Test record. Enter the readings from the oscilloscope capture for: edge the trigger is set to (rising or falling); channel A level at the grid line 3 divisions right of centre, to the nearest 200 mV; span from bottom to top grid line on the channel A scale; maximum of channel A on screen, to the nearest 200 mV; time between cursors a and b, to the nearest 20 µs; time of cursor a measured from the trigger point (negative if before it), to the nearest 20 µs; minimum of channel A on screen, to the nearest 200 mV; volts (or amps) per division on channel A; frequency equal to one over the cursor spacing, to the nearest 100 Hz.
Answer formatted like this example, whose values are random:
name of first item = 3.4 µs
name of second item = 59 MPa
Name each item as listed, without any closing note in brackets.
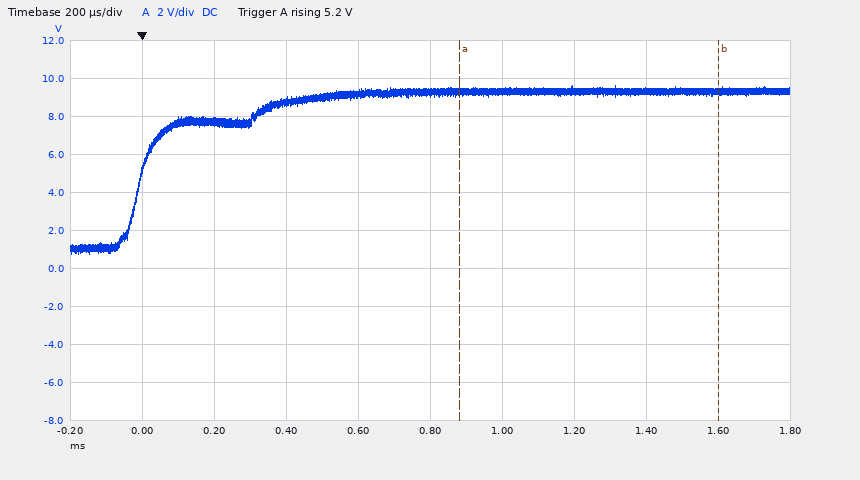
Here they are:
edge the trigger is set to = rising
channel A level at the grid line 3 divisions right of centre, to the nearest 200 mV = 9.4 V
span from bottom to top grid line on the channel A scale = 20 V
maximum of channel A on screen, to the nearest 200 mV = 9.6 V
time between cursors a and b, to the nearest 20 µs = 720 µs
time of cursor a measured from the trigger point (negative if before it), to the nearest 20 µs = +880 µs
minimum of channel A on screen, to the nearest 200 mV = 800 mV
volts (or amps) per division on channel A = 2 V
frequency equal to one over the cursor spacing, to the nearest 100 Hz = 1.4 kHz
